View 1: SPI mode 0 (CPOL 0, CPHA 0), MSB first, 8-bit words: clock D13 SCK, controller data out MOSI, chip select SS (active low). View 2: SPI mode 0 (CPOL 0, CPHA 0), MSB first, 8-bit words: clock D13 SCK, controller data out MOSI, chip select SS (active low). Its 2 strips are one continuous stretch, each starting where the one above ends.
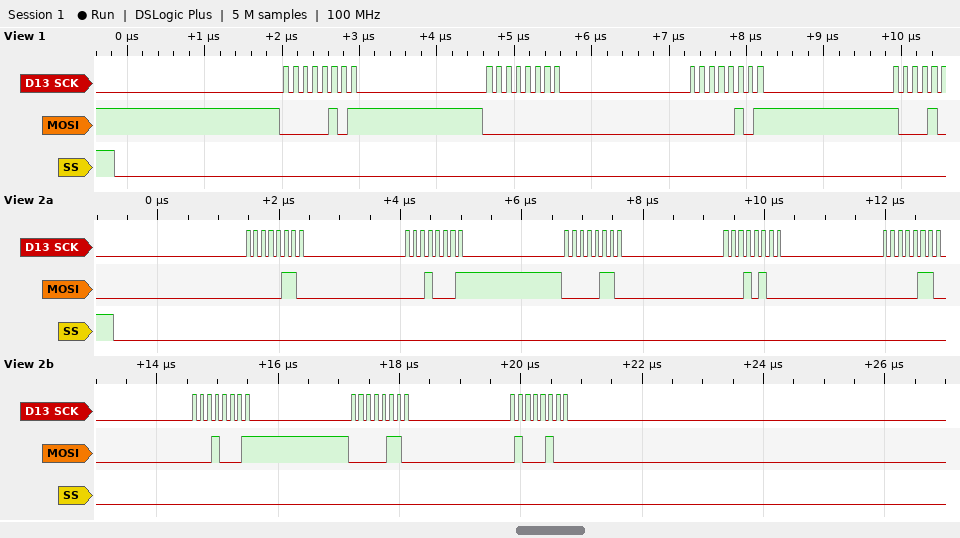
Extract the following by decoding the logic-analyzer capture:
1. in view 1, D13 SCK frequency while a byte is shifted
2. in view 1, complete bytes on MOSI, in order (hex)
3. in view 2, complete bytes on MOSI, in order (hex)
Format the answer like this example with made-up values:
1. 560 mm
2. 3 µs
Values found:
1. 8 MHz
2. 0x05 0x00 0x05
3. 06 11 06 14 06 11 06 44
